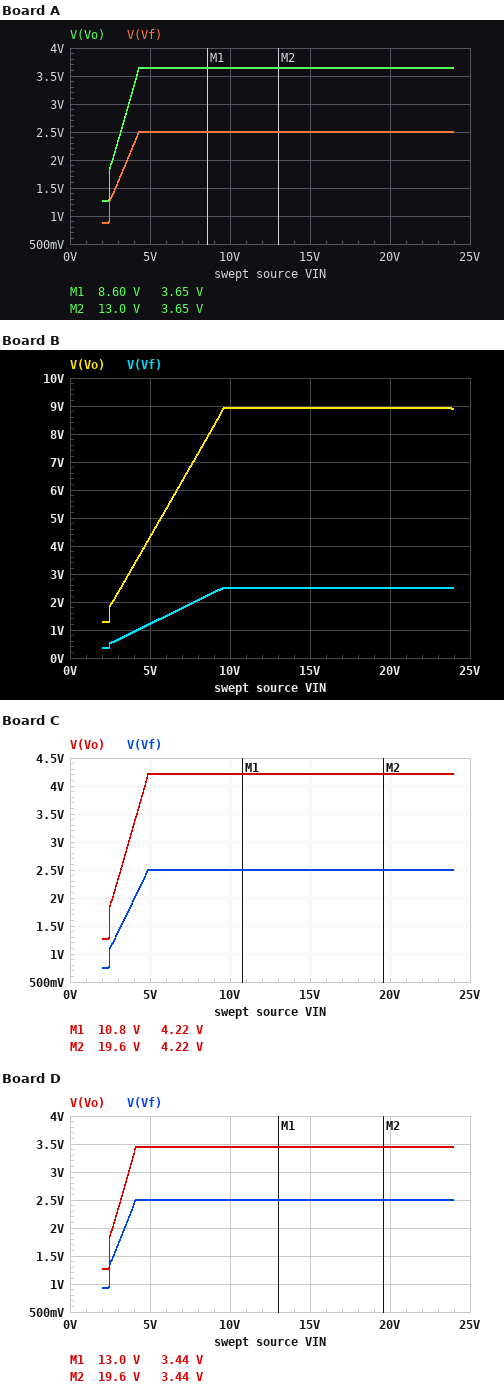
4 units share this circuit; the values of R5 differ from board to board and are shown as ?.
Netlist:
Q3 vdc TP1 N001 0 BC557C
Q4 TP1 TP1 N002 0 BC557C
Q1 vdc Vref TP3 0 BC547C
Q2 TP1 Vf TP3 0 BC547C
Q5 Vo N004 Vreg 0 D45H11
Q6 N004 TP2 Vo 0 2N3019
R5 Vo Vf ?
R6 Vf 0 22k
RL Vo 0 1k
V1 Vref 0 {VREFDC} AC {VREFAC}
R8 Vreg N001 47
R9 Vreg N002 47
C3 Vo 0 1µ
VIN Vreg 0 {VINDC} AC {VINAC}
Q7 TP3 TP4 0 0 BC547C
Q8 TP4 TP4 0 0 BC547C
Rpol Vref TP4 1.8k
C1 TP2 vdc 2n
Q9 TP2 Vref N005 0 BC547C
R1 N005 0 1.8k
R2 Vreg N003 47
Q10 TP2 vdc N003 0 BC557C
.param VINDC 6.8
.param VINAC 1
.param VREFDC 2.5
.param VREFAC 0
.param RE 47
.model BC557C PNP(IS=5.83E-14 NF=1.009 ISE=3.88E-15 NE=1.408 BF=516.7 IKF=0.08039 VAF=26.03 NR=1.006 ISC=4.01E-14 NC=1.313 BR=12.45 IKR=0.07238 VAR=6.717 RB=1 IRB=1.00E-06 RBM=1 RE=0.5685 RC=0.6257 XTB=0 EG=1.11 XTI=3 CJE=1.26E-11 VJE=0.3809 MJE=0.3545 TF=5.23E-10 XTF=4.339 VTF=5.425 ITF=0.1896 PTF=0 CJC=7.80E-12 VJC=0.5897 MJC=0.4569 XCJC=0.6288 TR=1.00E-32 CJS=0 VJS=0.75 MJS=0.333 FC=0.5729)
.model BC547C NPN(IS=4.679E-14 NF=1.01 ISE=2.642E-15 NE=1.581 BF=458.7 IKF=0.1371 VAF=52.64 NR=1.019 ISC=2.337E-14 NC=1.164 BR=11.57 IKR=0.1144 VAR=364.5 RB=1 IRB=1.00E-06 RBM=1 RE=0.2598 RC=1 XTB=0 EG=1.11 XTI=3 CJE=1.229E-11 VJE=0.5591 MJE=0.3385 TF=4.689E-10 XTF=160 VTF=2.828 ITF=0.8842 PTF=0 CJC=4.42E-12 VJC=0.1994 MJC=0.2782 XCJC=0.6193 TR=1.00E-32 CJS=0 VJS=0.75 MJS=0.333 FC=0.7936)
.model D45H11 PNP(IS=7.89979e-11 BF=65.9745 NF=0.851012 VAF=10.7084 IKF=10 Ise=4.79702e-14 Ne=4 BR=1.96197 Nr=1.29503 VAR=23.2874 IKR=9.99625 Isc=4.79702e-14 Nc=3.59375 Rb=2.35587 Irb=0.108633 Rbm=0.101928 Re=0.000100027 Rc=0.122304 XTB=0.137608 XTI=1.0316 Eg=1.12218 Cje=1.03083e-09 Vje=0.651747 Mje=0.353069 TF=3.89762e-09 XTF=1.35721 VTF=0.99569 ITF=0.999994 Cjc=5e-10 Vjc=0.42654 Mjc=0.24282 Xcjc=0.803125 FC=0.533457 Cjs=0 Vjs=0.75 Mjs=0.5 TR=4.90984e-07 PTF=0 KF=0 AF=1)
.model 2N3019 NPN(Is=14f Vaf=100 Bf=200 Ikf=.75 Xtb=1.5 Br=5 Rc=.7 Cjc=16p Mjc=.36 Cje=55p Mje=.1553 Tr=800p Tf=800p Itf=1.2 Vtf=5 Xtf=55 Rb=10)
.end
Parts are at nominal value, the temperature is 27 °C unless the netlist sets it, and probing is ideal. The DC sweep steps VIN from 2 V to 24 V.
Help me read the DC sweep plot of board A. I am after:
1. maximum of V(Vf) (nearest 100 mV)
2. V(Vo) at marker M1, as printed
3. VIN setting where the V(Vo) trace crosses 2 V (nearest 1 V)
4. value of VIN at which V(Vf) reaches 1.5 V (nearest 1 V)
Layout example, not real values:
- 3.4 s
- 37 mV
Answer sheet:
- 2.5 V
- 3.65 V
- 3 V
- 3 V
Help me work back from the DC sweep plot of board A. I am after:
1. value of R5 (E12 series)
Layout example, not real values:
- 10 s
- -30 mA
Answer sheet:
- 10 kΩ
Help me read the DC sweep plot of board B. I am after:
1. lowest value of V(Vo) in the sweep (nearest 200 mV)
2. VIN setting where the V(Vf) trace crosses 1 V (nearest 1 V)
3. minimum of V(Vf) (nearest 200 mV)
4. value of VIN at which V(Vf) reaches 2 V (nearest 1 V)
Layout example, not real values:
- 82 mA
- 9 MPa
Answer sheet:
- 1.2 V
- 4 V
- 400 mV
- 8 V
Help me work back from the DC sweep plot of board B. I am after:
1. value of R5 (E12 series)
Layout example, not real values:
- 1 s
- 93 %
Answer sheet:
- 56 kΩ
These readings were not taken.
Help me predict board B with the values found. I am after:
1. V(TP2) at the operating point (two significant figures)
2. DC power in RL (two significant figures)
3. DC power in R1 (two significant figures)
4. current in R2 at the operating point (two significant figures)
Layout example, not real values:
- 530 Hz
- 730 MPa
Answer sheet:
- 6.7 V
- 37 mW
- 2.0 mW
- 2.1 mA
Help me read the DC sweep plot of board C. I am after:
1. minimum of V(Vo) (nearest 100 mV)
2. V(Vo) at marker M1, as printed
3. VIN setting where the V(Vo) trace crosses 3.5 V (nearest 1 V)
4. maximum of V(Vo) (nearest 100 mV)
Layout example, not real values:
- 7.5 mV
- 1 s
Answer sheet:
- 1.3 V
- 4.22 V
- 4 V
- 4.2 V
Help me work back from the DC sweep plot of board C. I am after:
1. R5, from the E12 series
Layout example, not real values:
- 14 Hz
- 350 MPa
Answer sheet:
- 15 kΩ
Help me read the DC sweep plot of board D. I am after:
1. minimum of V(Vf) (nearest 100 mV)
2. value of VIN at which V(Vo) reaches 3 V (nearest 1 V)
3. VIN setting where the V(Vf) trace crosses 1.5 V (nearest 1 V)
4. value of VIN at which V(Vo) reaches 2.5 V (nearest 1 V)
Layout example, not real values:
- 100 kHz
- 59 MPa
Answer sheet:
- 900 mV
- 4 V
- 3 V
- 3 V
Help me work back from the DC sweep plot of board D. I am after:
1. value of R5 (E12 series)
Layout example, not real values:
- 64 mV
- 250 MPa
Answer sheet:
- 8.2 kΩ
